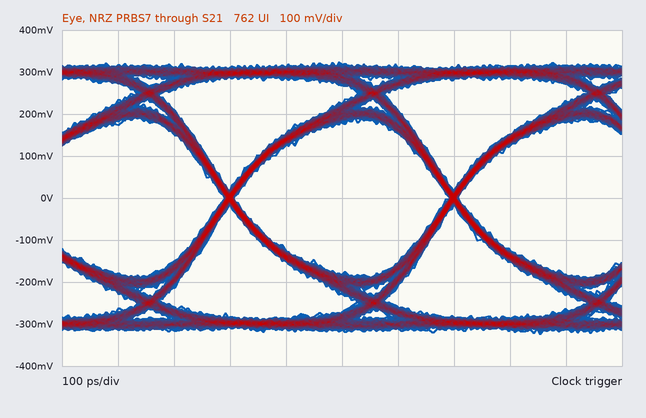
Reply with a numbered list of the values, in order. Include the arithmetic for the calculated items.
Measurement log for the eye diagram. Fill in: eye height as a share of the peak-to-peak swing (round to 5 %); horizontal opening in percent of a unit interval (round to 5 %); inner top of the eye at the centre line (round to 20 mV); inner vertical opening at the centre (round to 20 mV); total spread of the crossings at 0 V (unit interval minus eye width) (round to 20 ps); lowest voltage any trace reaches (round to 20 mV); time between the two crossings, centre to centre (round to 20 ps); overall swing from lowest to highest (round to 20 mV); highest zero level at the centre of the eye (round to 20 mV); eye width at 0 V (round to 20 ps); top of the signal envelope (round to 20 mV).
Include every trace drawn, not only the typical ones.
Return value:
1. 360 mV / 640 mV ≈ 56.2 %, so 55 % to the nearest 5 %
2. 380 ps / 400 ps ≈ 95 %
3. 180 mV
4. 360 mV
5. 20 ps
6. -320 mV
7. 400 ps
8. 640 mV
9. -180 mV
10. 380 ps
11. 320 mV
